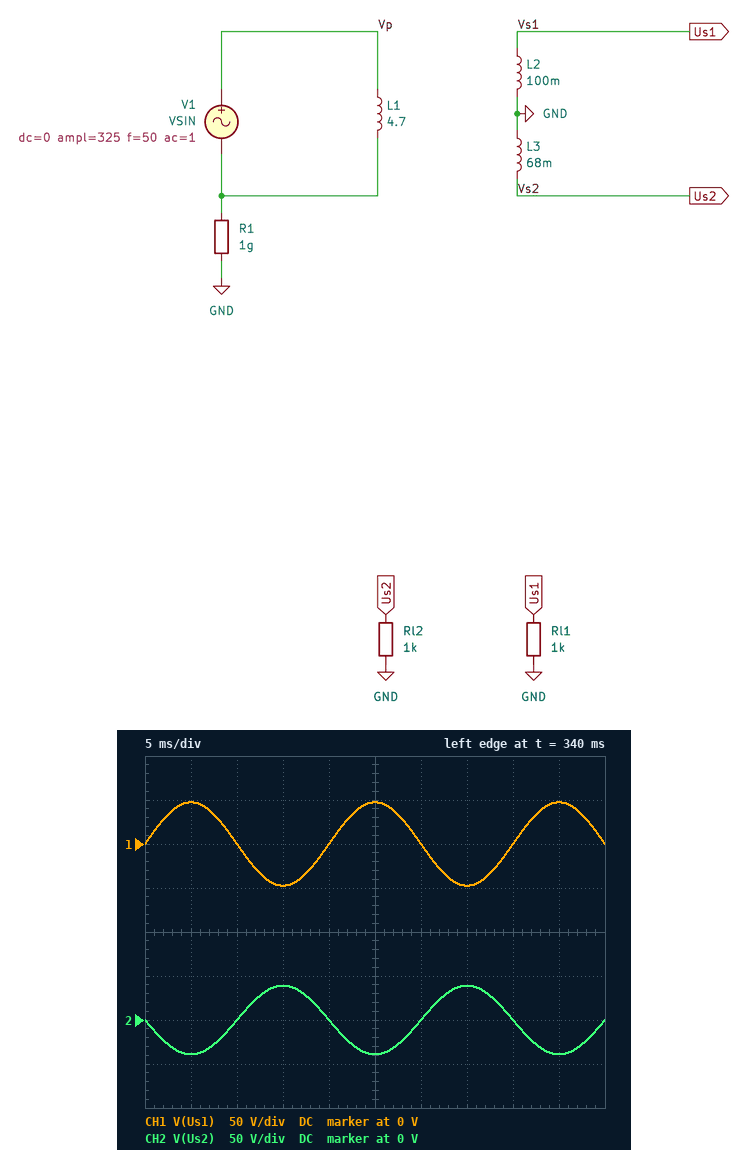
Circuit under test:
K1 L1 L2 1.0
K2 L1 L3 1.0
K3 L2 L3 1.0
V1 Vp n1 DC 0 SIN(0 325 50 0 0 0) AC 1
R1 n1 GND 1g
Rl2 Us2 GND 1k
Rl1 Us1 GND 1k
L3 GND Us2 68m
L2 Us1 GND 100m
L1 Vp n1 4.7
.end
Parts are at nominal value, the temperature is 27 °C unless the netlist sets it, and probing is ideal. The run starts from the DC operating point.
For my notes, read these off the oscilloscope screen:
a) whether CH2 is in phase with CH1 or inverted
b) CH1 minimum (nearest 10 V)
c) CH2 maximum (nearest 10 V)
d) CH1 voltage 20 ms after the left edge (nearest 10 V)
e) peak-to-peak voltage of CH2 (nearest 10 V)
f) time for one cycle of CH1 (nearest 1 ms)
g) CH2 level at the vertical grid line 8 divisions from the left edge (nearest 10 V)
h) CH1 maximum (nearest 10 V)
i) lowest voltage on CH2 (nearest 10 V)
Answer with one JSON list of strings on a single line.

["inverted", "-50 V", "40 V", "0 V", "80 V", "20 ms", "0 V", "50 V", "-40 V"]
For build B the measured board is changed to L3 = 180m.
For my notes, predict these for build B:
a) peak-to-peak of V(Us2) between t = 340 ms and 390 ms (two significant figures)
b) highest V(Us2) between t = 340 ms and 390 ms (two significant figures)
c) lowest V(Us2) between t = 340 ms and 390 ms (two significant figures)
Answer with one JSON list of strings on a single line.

["130 V", "64 V", "-64 V"]
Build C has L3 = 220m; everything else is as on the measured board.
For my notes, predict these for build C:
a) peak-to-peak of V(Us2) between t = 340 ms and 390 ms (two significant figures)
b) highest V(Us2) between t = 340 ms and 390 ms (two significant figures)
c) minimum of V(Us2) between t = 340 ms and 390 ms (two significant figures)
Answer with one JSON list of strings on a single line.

["140 V", "70 V", "-70 V"]
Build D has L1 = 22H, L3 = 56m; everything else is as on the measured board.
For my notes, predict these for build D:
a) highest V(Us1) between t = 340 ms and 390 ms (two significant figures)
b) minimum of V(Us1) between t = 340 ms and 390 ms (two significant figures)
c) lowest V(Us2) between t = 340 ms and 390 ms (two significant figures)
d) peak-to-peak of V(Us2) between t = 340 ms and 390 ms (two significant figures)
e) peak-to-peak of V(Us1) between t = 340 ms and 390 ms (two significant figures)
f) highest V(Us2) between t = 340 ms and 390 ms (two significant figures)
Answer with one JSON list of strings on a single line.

["22 V", "-22 V", "-16 V", "33 V", "44 V", "16 V"]
